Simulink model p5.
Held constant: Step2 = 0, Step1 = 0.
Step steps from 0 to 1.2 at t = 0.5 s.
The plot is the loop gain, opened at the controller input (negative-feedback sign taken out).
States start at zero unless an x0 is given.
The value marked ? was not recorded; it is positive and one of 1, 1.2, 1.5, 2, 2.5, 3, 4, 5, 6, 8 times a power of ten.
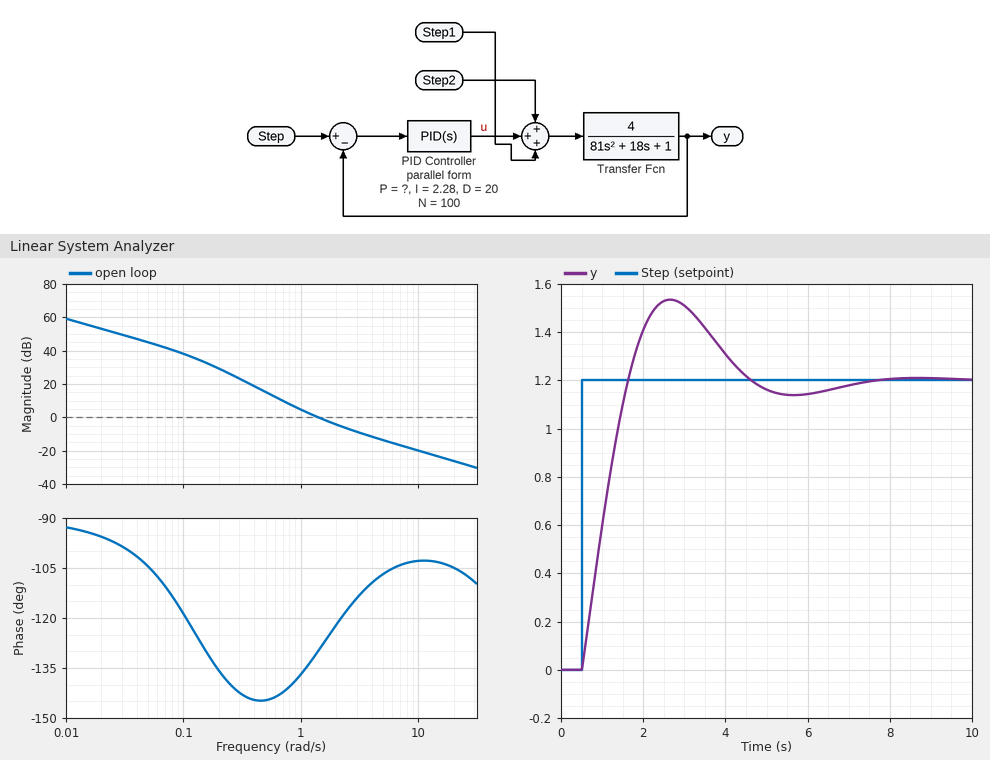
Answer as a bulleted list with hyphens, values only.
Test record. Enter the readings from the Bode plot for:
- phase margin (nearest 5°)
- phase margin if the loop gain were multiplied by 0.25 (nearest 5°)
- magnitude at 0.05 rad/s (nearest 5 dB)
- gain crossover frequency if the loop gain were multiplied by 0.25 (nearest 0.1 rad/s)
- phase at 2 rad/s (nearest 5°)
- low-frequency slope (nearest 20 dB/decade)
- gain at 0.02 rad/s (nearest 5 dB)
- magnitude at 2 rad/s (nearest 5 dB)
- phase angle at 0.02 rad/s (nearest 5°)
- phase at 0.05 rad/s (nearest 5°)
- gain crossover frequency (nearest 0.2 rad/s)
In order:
- 50°
- 35°
- 45 dB
- 0.6 rad/s
- -120°
- -20 dB/decade
- 55 dB
- -5 dB
- -95°
- -105°
- 1.4 rad/s
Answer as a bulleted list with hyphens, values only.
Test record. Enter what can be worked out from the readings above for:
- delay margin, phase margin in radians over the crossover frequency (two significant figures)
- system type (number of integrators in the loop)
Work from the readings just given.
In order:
- 0.62 s
- 1
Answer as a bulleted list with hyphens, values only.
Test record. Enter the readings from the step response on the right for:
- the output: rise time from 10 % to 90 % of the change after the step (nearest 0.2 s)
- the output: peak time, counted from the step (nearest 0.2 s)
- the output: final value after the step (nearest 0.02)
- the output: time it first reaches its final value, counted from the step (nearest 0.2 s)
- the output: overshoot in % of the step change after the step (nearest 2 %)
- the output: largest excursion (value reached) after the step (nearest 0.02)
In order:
- 0.8 s
- 2.2 s
- 1.20
- 1.2 s
- 28 %
- 1.54
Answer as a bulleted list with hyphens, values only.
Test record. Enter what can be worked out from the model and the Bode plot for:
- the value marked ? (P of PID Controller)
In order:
- 30
